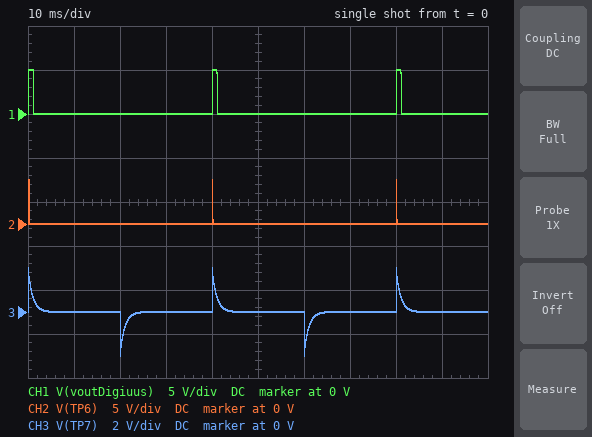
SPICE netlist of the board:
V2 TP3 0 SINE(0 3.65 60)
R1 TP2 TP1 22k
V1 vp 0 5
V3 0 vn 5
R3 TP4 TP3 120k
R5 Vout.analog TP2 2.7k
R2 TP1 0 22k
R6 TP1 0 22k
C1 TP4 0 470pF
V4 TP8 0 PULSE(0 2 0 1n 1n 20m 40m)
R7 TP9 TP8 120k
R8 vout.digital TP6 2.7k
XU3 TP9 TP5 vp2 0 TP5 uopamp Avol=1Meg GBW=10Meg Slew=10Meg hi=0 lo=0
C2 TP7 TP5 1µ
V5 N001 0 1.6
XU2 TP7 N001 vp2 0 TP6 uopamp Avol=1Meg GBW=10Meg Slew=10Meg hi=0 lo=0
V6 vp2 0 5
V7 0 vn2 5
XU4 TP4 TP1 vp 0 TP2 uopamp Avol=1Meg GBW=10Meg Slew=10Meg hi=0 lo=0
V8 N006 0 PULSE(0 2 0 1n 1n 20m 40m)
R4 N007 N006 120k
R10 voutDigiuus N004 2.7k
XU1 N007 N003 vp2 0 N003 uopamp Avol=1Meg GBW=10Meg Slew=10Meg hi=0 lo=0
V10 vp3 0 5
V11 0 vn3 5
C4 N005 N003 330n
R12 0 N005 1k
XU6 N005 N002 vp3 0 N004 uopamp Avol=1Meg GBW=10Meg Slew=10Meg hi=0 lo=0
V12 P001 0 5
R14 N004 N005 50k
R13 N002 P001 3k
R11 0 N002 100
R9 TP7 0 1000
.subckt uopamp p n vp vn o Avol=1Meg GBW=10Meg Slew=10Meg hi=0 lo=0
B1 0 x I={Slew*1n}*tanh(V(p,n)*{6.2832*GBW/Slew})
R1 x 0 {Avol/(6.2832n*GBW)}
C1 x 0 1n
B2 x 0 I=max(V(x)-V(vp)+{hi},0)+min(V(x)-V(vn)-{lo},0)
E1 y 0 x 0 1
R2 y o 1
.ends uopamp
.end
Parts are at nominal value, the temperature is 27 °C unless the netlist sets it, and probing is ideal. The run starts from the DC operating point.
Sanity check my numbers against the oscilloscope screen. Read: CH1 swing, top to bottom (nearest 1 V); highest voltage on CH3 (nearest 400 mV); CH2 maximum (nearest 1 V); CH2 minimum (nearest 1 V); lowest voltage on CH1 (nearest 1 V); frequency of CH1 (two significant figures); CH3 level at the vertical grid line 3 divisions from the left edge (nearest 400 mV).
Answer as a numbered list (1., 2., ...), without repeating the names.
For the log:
1. 5 V
2. 2.0 V
3. 5 V
4. 0 V
5. 0 V
6. 25 Hz
7. 0 V
